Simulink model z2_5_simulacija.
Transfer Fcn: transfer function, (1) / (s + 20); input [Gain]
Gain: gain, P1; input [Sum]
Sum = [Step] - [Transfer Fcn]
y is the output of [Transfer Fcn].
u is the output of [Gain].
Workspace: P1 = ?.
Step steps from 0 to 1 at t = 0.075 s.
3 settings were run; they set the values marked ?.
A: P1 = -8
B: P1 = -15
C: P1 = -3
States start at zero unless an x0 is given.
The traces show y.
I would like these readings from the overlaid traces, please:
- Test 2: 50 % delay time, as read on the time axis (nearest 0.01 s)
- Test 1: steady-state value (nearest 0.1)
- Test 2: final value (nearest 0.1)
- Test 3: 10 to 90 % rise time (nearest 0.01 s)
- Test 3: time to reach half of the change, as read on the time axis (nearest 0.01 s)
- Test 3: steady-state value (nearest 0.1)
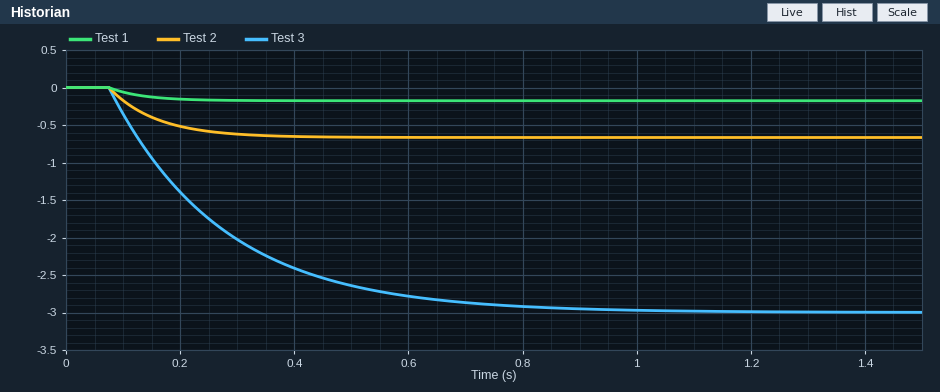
0.13 s
-0.2
-0.7
0.44 s
0.21 s
-3.0
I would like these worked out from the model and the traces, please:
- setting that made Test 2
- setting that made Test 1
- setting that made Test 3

A
C
B
